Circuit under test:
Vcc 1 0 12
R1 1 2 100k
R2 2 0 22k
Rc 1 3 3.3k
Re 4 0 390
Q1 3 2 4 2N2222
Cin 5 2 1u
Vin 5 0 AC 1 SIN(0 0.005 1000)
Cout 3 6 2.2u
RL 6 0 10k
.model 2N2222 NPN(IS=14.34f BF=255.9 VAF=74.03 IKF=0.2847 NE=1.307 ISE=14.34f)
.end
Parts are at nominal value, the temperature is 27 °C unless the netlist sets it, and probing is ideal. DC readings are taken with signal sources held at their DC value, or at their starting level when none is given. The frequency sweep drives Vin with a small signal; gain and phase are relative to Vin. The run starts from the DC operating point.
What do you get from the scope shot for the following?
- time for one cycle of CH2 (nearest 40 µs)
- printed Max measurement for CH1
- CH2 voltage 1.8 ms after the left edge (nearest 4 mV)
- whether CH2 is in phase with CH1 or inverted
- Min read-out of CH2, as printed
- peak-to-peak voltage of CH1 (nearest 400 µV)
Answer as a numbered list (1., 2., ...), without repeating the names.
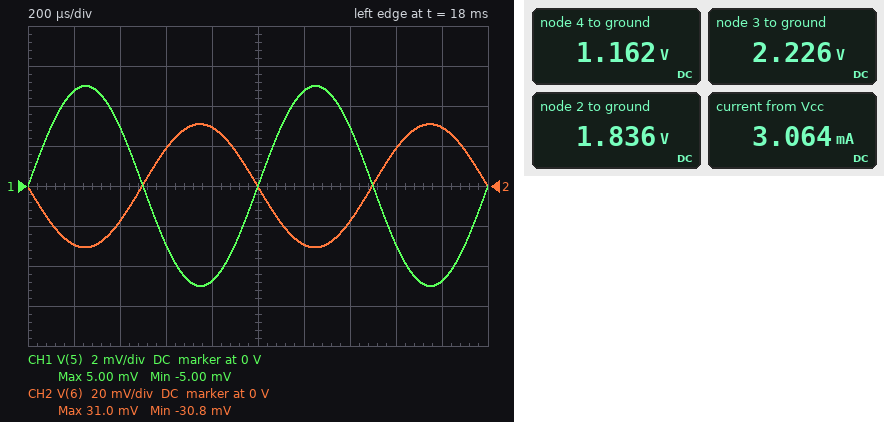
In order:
1. 1.00 ms
2. 5.00 mV
3. 28 mV
4. inverted
5. -30.8 mV
6. 10.0 mV
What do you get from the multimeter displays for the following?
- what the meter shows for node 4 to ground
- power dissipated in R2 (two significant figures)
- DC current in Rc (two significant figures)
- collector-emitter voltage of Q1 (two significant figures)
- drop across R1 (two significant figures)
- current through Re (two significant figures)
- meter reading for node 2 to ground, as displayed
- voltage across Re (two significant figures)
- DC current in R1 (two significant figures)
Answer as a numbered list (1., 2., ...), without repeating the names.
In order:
1. 1.162 V
2. 150 µW
3. 3.0 mA
4. 1.1 V
5. 10 V
6. 3.0 mA
7. 1.836 V
8. 1.2 V
9. 100 µA
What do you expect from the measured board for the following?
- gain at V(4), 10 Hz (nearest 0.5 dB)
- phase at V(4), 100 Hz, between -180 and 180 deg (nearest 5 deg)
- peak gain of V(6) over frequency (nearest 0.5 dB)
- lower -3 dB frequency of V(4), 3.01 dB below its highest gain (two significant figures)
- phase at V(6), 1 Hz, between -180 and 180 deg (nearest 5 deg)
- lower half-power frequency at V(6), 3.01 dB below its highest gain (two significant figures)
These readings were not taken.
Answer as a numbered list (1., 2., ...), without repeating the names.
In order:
1. -4.0 dB
2. 5 deg
3. 16.0 dB
4. 11 Hz
5. -15 deg
6. 13 Hz
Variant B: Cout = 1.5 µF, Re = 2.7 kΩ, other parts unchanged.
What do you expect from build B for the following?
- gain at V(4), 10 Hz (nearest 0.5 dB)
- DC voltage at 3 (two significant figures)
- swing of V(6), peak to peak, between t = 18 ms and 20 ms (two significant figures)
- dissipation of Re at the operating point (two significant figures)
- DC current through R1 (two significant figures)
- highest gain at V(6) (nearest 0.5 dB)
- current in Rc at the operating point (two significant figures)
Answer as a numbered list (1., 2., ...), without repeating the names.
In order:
1. -3.0 dB
2. 10 V
3. 9.0 mV
4. 800 µW
5. 99 µA
6. -1.0 dB
7. 540 µA
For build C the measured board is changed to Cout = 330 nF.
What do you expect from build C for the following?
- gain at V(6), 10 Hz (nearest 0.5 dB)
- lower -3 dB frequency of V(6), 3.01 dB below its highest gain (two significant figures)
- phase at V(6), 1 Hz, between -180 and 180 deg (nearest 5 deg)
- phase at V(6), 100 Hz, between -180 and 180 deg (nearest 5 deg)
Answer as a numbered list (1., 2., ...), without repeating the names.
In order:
1. 0.5 dB
2. 39 Hz
3. -5 deg
4. -155 deg
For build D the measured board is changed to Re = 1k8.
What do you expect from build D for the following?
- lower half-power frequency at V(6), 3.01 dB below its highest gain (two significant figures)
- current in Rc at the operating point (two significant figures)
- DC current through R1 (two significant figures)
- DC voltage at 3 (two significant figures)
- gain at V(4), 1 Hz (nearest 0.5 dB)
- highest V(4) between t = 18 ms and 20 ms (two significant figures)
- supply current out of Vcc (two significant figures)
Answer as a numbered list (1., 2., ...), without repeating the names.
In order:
1. 12 Hz
2. 790 µA
3. 99 µA
4. 9.4 V
5. -19.5 dB
6. 1.4 V
7. 890 µA
